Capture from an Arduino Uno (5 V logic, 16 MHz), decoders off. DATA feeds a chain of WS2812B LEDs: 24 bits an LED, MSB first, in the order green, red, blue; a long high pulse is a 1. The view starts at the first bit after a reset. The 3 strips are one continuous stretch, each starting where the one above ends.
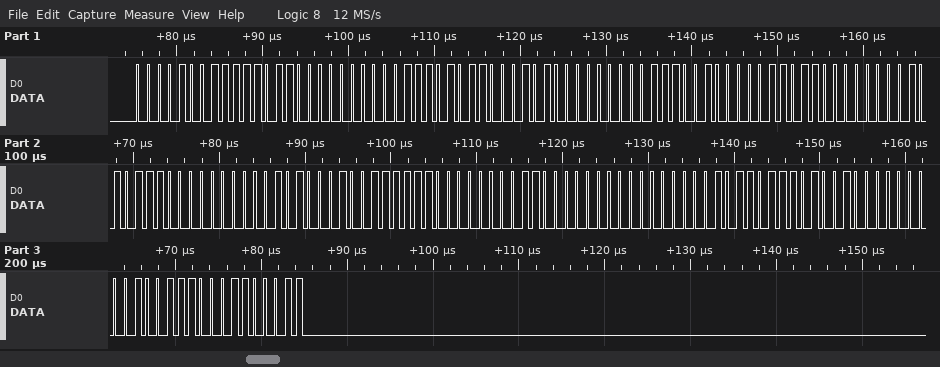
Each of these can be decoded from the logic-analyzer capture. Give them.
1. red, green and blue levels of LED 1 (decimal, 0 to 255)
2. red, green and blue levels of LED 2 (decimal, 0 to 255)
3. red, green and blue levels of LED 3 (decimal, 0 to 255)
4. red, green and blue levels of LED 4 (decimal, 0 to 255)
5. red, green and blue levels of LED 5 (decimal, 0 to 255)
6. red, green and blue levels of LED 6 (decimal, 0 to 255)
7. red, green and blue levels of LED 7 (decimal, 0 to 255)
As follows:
246, 9, 0
138, 117, 0
27, 228, 0
0, 174, 81
0, 63, 192
45, 0, 210
156, 0, 99
